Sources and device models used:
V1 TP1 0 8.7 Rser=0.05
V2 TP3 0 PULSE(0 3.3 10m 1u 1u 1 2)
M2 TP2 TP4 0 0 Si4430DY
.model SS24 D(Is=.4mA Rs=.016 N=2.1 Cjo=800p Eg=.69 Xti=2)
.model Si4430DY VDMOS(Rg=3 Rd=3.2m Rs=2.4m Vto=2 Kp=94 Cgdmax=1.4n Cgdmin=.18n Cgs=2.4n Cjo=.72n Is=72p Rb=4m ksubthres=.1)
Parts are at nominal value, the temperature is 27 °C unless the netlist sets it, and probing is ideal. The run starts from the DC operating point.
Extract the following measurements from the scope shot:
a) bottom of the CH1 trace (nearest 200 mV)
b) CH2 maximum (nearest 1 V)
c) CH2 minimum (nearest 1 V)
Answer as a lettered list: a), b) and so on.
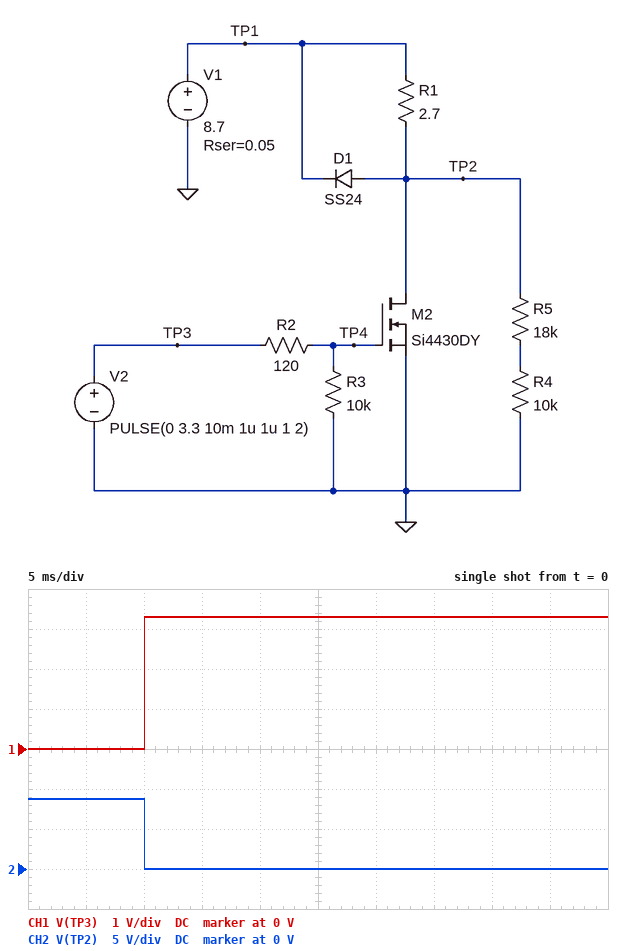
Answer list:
a) 0 V
b) 9 V
c) 0 V
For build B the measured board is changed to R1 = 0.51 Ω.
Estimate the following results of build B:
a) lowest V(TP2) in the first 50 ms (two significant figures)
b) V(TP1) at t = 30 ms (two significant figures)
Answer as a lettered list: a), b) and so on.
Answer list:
a) 220 mV
b) 7.9 V
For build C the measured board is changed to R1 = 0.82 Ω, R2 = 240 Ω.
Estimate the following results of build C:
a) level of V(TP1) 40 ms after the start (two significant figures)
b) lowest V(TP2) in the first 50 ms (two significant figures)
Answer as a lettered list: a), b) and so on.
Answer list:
a) 8.2 V
b) 150 mV
